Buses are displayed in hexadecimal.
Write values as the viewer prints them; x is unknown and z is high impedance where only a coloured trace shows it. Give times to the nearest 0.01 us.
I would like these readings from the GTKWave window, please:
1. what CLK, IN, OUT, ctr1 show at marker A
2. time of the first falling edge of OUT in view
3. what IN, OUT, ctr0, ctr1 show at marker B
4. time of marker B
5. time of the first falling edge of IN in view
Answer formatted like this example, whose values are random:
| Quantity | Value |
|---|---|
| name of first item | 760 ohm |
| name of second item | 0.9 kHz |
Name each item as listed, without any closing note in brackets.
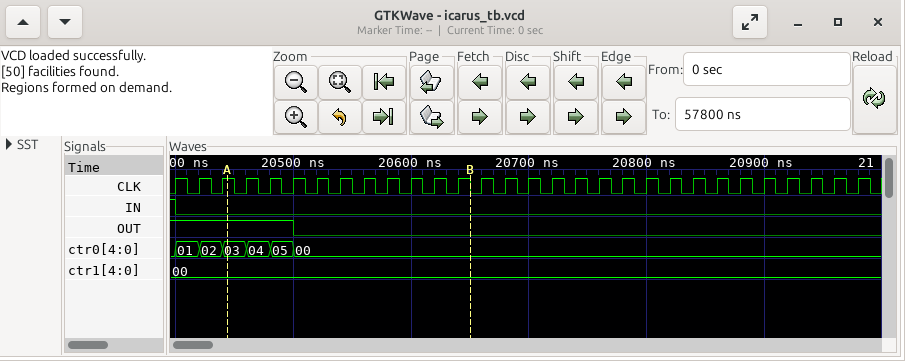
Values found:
| Quantity | Value |
|---|---|
| what CLK, IN, OUT, ctr1 show at marker A | CLK=1, IN=0, OUT=1, ctr1=00 |
| time of the first falling edge of OUT in view | 20.5 us |
| what IN, OUT, ctr0, ctr1 show at marker B | IN=0, OUT=0, ctr0=00, ctr1=00 |
| time of marker B | 20.65 us |
| time of the first falling edge of IN in view | 20.4 us |
